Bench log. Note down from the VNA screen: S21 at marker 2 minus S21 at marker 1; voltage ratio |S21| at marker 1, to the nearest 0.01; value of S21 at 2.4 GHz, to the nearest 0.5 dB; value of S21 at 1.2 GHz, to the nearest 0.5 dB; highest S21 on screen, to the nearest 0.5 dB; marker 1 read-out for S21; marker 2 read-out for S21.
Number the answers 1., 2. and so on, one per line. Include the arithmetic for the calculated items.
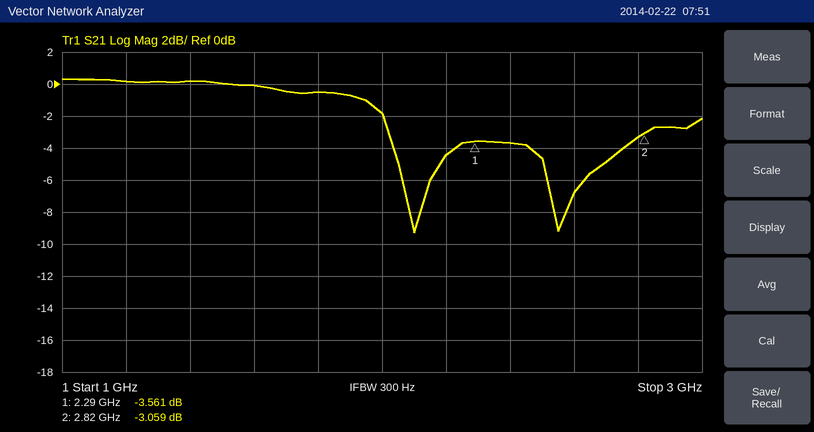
1. -3.059 − (-3.561) = 0.502 dB
2. 10^(-3.561/20) ≈ 0.66
3. -3.5 dB
4. 0.0 dB
5. 0.5 dB
6. -3.561 dB
7. -3.059 dB
